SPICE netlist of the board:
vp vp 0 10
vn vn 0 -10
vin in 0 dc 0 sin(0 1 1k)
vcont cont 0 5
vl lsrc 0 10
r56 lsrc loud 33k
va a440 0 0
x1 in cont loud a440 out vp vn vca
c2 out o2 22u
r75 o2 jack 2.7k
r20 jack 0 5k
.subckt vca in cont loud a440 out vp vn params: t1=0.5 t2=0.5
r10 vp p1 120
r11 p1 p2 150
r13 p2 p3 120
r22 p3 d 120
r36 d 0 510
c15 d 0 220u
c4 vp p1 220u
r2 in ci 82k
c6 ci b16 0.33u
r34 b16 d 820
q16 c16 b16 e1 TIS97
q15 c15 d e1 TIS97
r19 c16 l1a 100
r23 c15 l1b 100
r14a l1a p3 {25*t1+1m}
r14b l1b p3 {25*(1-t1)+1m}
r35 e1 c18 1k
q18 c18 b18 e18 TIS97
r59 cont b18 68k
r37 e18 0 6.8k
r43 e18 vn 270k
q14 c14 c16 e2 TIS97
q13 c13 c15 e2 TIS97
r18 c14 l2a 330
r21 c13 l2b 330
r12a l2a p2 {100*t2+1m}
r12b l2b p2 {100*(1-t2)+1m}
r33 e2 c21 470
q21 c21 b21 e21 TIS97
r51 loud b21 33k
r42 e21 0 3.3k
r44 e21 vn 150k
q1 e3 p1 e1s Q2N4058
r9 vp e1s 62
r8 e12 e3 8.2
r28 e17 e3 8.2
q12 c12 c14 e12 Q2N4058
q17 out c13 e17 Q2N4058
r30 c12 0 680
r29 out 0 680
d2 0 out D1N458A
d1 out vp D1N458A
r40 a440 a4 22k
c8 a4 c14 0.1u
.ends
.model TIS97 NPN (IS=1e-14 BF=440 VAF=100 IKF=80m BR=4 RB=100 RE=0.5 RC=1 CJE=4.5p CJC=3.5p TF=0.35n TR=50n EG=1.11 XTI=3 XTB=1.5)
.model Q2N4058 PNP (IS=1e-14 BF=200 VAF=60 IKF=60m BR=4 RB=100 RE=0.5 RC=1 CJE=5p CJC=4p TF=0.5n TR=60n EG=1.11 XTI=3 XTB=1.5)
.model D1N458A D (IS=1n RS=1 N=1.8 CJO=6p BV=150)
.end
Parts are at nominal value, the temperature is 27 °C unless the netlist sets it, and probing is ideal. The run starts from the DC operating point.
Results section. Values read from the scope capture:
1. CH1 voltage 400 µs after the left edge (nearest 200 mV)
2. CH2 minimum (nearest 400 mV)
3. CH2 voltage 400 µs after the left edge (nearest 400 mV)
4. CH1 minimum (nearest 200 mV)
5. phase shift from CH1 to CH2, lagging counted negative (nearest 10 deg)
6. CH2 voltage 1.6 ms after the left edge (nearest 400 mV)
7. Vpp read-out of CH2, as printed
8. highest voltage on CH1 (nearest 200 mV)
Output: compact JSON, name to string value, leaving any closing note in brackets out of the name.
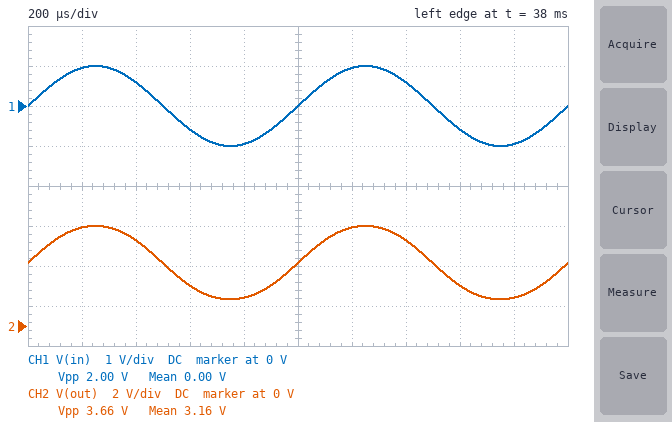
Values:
{"CH1 voltage 400 µs after the left edge": "600 mV", "CH2 minimum": "1.2 V", "CH2 voltage 400 µs after the left edge": "4.4 V", "CH1 minimum": "-1.0 V", "phase shift from CH1 to CH2, lagging counted negative": "0 deg", "CH2 voltage 1.6 ms after the left edge": "2.0 V", "Vpp read-out of CH2, as printed": "3.66 V", "highest voltage on CH1": "1.0 V"}
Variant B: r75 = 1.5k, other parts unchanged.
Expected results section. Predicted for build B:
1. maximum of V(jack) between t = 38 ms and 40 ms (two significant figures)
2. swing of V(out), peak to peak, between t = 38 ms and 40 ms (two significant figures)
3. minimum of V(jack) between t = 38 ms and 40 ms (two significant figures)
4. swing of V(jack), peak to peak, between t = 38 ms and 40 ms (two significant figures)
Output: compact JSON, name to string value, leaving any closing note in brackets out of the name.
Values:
{"maximum of V(jack) between t = 38 ms and 40 ms": "1.4 V", "swing of V(out), peak to peak, between t = 38 ms and 40 ms": "3.6 V", "minimum of V(jack) between t = 38 ms and 40 ms": "-1.4 V", "swing of V(jack), peak to peak, between t = 38 ms and 40 ms": "2.8 V"}
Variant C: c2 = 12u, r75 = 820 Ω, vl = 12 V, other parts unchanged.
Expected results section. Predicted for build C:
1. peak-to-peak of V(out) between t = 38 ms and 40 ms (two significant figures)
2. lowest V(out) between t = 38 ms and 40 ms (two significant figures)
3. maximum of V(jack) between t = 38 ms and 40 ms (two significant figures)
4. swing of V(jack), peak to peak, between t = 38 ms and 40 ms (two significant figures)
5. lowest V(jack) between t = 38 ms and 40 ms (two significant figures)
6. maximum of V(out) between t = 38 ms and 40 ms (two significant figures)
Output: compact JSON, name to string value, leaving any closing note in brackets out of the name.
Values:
{"peak-to-peak of V(out) between t = 38 ms and 40 ms": "3.5 V", "lowest V(out) between t = 38 ms and 40 ms": "1.4 V", "maximum of V(jack) between t = 38 ms and 40 ms": "1.5 V", "swing of V(jack), peak to peak, between t = 38 ms and 40 ms": "3.0 V", "lowest V(jack) between t = 38 ms and 40 ms": "-1.5 V", "maximum of V(out) between t = 38 ms and 40 ms": "4.9 V"}
